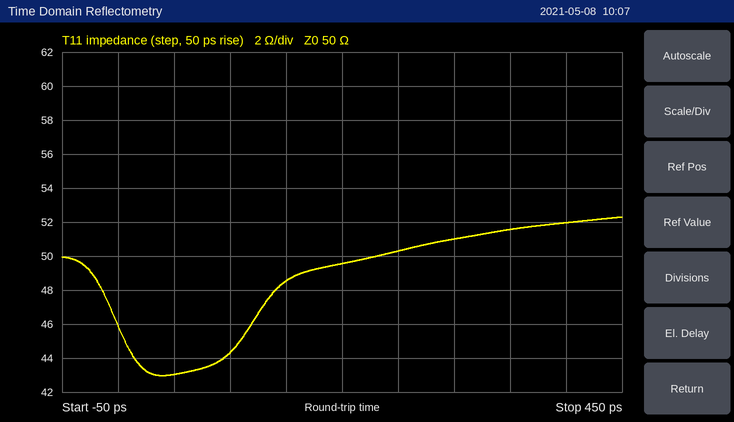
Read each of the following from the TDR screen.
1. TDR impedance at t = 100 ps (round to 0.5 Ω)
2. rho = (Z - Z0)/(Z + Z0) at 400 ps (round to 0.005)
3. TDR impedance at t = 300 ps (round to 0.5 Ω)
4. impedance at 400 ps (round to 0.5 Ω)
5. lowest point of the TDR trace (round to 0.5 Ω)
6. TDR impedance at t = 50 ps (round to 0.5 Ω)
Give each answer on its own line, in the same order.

44.5 Ω
+0.020
51.0 Ω
52.0 Ω
43.0 Ω
43.0 Ω
